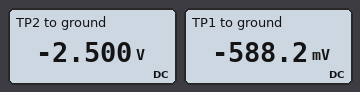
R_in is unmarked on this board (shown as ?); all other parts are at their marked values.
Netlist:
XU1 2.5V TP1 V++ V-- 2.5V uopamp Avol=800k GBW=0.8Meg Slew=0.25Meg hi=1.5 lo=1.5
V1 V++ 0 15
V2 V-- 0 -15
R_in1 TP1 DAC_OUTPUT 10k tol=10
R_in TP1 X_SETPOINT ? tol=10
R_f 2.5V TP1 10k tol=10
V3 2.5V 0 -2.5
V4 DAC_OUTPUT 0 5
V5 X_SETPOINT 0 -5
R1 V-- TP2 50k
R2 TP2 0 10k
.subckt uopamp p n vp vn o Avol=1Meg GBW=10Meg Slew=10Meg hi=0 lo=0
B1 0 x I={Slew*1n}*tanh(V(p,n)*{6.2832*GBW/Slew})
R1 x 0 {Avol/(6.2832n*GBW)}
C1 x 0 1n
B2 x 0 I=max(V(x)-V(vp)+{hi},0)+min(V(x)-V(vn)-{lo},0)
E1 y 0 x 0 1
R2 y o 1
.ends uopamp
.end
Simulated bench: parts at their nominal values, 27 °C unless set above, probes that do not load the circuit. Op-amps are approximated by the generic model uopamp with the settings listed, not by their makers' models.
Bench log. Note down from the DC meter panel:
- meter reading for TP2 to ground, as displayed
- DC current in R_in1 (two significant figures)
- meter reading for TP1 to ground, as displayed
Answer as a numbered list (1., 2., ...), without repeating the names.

1. -2.500 V
2. 560 µA
3. -588.2 mV
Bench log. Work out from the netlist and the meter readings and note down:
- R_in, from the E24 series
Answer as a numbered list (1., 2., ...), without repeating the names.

1. 12 kΩ
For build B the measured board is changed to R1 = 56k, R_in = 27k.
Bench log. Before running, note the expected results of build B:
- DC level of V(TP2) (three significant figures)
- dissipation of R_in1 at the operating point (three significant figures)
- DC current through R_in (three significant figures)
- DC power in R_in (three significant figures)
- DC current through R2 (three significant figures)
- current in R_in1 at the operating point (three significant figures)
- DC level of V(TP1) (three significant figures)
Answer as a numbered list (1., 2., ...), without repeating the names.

1. -2.27 V
2. 2.23 mW
3. 195 µA
4. 1.03 mW
5. 227 µA
6. 473 µA
7. 273 mV
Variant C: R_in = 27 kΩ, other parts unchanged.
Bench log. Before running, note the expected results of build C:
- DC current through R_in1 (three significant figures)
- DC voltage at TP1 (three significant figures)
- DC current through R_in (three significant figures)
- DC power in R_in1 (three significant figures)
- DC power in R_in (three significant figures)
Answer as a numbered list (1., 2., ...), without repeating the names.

1. 473 µA
2. 273 mV
3. 195 µA
4. 2.23 mW
5. 1.03 mW
